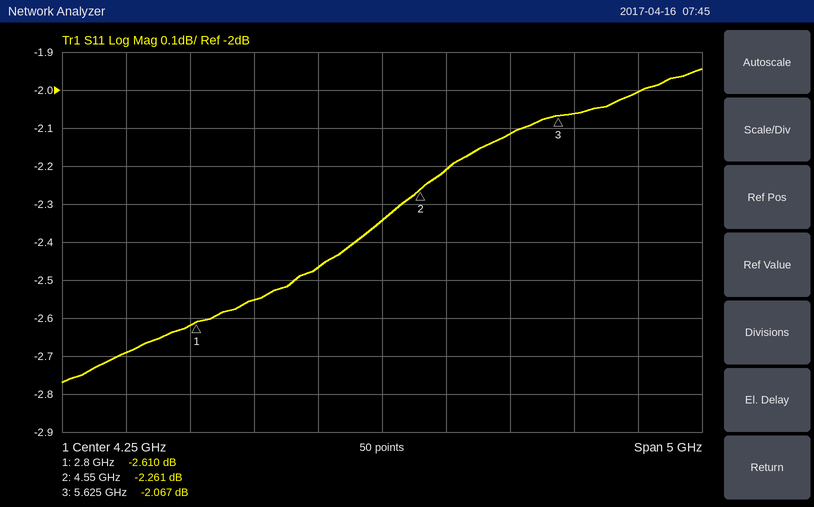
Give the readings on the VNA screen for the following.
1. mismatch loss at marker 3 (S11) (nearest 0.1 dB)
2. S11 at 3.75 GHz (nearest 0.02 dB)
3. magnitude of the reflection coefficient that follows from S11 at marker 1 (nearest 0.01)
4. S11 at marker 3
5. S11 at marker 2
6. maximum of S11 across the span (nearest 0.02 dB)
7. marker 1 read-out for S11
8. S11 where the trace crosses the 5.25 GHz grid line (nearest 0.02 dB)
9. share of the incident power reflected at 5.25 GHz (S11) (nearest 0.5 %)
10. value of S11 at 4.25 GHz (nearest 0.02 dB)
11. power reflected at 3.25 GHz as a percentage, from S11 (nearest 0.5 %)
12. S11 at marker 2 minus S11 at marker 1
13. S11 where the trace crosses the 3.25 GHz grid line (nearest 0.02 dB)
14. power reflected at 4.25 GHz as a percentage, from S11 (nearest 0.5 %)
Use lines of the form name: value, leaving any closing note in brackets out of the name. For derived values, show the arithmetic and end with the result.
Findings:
mismatch loss at marker 3 (S11): −10 log10(1 − 10^(-2.067/10)) ≈ 4.2 dB
S11 at 3.75 GHz: -2.46 dB
magnitude of the reflection coefficient that follows from S11 at marker 1: 10^(-2.61/20) ≈ 0.74
S11 at marker 3: -2.067 dB
S11 at marker 2: -2.261 dB
maximum of S11 across the span: -1.94 dB
marker 1 read-out for S11: -2.610 dB
S11 where the trace crosses the 5.25 GHz grid line: -2.12 dB
share of the incident power reflected at 5.25 GHz (S11): 10^(-2.12/10) ≈ 61.4 %, so 61.5 % to the nearest 0.5 %
value of S11 at 4.25 GHz: -2.34 dB
power reflected at 3.25 GHz as a percentage, from S11: 10^(-2.56/10) ≈ 55.5 %
S11 at marker 2 minus S11 at marker 1: -2.261 − (-2.61) = 0.349 dB
S11 where the trace crosses the 3.25 GHz grid line: -2.56 dB
power reflected at 4.25 GHz as a percentage, from S11: 10^(-2.34/10) ≈ 58.3 %, so 58.5 % to the nearest 0.5 %
